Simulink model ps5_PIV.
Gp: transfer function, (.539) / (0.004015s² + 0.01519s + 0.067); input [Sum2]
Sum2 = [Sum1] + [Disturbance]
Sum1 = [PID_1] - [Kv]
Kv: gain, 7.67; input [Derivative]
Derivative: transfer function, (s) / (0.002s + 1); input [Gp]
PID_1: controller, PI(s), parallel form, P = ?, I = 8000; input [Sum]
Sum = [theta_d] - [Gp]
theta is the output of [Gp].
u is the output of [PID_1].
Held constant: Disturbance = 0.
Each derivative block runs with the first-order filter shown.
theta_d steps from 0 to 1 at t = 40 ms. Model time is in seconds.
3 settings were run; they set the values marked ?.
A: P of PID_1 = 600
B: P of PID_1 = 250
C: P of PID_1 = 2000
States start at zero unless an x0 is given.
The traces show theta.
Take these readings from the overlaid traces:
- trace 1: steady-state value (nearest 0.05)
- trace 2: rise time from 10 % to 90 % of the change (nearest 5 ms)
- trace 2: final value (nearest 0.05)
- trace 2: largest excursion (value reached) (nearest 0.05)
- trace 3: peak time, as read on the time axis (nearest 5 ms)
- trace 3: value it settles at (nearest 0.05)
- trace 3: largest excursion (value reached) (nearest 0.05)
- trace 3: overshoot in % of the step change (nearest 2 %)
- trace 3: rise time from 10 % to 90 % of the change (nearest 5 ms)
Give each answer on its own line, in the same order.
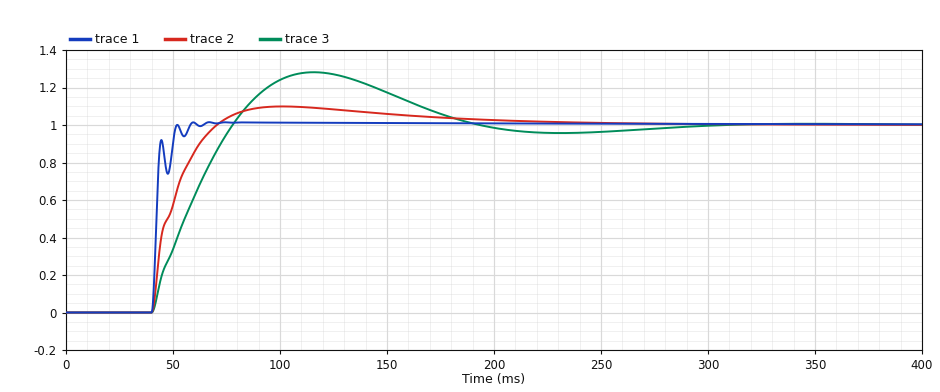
1.00
20 ms
1.00
1.10
115 ms
1.00
1.30
28 %
30 ms
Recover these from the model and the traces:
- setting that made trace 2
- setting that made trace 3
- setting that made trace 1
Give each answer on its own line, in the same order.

A
B
C
